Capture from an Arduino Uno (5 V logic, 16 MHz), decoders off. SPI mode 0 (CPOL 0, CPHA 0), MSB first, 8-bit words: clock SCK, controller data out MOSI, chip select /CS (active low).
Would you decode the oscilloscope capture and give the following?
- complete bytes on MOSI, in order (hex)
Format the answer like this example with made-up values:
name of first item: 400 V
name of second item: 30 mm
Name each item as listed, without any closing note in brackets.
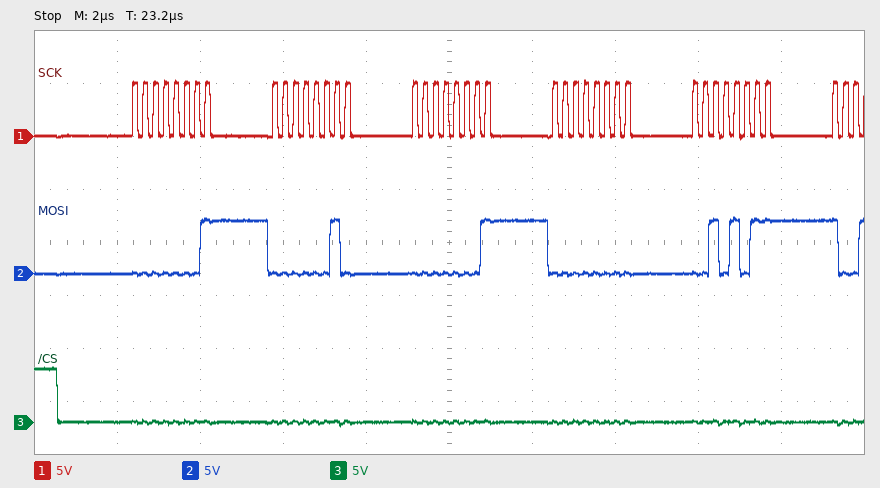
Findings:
complete bytes on MOSI, in order: 01 02 01 00 2B
